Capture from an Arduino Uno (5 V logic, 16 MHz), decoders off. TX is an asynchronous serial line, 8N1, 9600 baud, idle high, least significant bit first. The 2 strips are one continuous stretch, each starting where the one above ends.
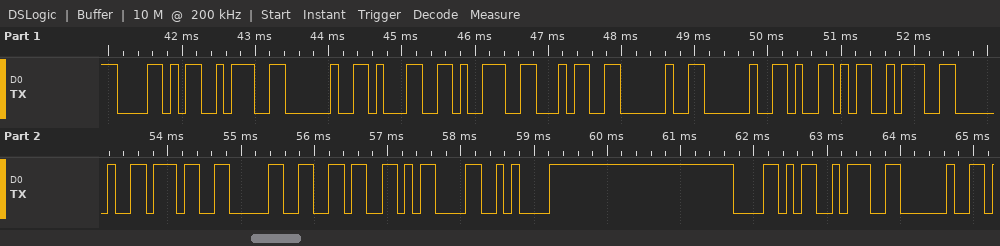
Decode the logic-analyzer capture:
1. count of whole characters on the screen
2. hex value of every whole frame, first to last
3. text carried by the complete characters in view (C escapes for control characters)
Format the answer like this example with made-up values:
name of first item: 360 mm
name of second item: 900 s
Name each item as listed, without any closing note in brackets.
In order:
count of whole characters on the screen: 19
hex value of every whole frame, first to last: 0x58 0x3A 0x20 0x31 0x39 0x34 0x20 0x20 0x59 0x3A 0x20 0x37 0x30 0x36 0x0D 0x0A 0x58 0x3A 0x20
text carried by the complete characters in view: "X: 194  Y: 706\r\nX: "
